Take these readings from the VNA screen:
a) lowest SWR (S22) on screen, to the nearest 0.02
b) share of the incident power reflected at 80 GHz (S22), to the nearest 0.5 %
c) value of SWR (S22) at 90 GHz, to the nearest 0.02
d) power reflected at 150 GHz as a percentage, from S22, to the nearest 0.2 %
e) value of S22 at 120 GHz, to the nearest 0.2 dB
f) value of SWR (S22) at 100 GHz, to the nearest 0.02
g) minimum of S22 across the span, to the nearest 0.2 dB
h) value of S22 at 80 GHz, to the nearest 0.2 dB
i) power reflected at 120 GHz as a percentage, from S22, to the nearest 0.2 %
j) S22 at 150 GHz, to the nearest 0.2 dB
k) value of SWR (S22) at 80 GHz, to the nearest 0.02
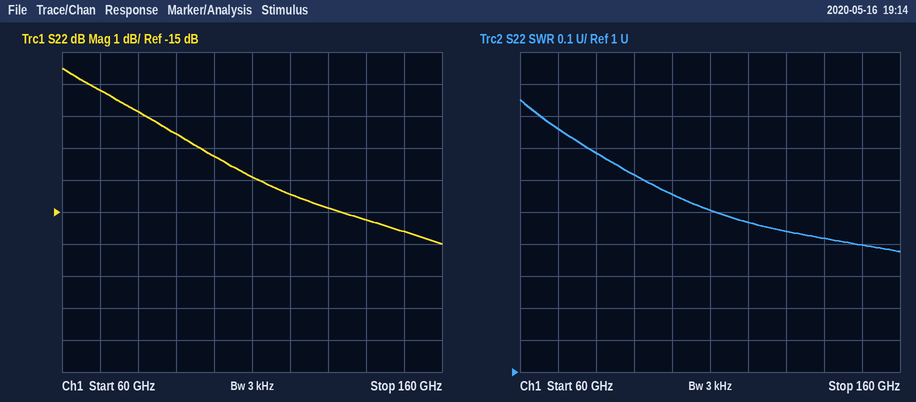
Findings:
1.38
6.5 %
1.62
2.8 %
-14.4 dB
1.56
-16.0 dB
-11.8 dB
3.6 %
-15.6 dB
1.68
